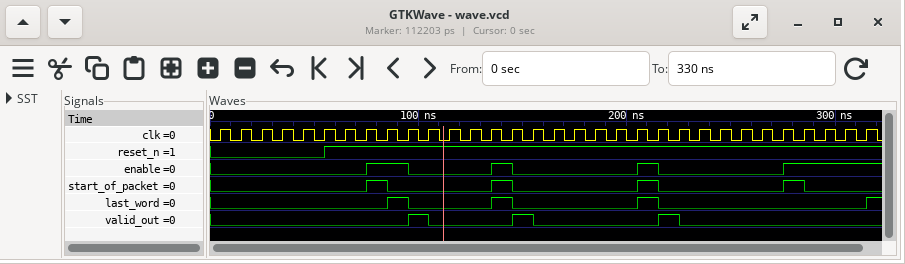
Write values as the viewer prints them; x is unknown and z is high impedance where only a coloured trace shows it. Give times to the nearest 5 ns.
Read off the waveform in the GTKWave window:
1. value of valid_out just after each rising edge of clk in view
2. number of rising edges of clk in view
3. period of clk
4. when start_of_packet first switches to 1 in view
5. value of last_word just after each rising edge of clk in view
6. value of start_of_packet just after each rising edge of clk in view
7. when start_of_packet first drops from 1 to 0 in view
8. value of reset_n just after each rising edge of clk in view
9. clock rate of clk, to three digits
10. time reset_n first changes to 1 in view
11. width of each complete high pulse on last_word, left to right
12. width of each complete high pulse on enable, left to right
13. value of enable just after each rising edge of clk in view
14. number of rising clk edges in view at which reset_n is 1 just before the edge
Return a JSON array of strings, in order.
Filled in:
["0 0 0 0 0 0 0 0 0 1 0 0 0 0 1 0 0 0 0 0 0 1 0 0 0 0 0 0 0 0 0 0", "32", "10 ns", "75 ns", "0 0 0 0 0 0 0 0 1 0 0 0 0 1 0 0 0 0 0 0 1 0 0 0 0 0 0 0 0 0 0 1", "0 0 0 0 0 0 0 1 0 0 0 0 0 1 0 0 0 0 0 0 1 0 0 0 0 0 0 1 0 0 0 0", "85 ns", "0 0 0 0 0 1 1 1 1 1 1 1 1 1 1 1 1 1 1 1 1 1 1 1 1 1 1 1 1 1 1 1", "100 MHz", "55 ns", "10 ns, 10 ns, 10 ns", "20 ns, 10 ns, 10 ns", "0 0 0 0 0 0 0 1 1 0 0 0 0 1 0 0 0 0 0 0 1 0 0 0 0 0 0 1 1 1 1 1", "26"]
